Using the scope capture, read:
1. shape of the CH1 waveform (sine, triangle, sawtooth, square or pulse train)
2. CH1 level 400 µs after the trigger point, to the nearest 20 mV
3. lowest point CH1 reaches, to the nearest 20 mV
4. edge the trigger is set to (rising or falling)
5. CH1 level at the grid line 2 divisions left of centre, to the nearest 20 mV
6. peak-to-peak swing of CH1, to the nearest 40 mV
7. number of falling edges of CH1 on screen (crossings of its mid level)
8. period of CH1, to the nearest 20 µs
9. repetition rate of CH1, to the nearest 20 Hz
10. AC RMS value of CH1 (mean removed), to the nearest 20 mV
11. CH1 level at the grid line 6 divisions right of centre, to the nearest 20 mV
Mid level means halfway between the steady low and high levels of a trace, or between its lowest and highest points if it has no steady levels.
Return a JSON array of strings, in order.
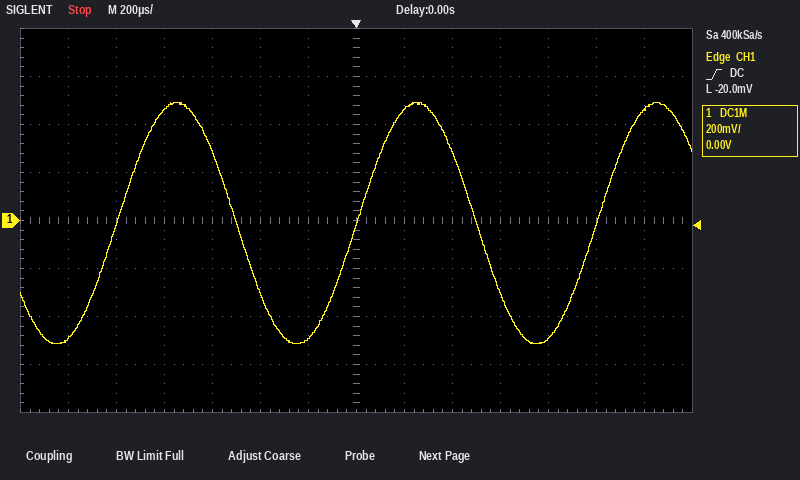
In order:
["sine", "280 mV", "-520 mV", "rising", "-300 mV", "1.00 V", "2", "1.00 ms", "1.00 kHz", "360 mV", "460 mV"]
